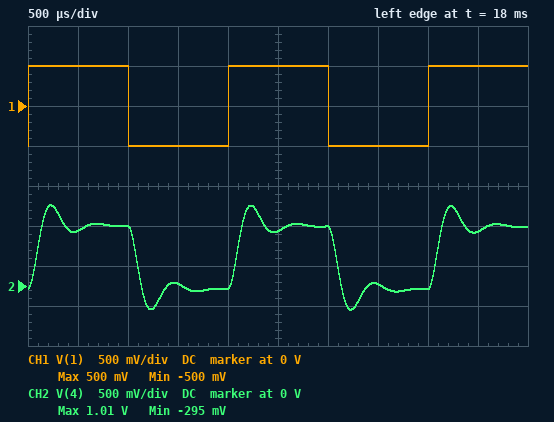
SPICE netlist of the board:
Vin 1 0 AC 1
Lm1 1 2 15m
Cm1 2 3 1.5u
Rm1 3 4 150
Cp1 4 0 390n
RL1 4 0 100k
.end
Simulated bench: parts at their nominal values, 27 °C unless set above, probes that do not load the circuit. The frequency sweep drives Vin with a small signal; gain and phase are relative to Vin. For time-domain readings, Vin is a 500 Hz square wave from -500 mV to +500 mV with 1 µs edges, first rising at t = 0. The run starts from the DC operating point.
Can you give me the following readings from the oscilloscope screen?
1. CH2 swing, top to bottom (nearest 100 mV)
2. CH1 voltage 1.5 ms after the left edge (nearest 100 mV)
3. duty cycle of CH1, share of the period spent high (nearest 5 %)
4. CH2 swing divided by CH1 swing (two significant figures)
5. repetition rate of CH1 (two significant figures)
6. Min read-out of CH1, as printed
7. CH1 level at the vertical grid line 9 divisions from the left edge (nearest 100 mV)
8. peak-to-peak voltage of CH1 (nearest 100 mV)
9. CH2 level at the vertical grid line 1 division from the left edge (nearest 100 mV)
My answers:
1.3 V
-500 mV
50 %
1.3
500 Hz
-500 mV
500 mV
1.0 V
700 mV
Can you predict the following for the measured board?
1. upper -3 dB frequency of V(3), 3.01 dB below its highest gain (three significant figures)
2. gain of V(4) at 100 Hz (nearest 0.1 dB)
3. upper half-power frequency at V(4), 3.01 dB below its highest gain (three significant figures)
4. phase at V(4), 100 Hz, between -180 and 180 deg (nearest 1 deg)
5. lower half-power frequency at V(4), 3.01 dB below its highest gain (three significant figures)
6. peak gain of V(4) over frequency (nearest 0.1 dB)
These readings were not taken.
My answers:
2.97 kHz
-2.0 dB
2.77 kHz
-1 deg
828 Hz
1.8 dB
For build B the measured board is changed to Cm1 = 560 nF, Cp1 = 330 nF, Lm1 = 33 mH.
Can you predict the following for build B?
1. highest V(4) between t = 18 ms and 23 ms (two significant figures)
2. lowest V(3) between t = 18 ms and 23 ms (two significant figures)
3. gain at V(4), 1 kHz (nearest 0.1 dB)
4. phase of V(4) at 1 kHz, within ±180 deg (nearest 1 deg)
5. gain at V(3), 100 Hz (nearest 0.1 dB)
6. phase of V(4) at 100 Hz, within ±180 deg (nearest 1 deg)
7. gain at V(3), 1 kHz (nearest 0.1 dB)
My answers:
890 mV
-450 mV
-1.6 dB
-15 deg
-4.0 dB
0 deg
-1.2 dB
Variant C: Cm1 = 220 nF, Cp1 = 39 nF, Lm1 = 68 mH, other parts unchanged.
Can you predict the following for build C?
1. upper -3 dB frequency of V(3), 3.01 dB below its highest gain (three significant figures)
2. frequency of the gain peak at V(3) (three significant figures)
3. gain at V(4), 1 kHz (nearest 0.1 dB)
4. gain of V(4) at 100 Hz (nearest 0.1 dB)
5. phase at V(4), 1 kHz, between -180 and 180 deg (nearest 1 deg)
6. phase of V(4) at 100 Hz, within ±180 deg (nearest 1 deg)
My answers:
3.53 kHz
3.34 kHz
-0.6 dB
-1.4 dB
-2 deg
3 deg
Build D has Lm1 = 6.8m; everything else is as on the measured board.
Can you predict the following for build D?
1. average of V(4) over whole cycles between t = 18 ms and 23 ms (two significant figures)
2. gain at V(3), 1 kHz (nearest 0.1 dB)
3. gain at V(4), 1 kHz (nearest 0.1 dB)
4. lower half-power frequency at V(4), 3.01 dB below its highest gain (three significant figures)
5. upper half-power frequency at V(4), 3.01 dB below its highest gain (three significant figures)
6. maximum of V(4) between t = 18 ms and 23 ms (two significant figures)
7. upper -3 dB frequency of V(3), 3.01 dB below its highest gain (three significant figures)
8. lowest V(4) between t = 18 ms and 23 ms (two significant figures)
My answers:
360 mV
-1.1 dB
-1.7 dB
1.16 Hz
4.05 kHz
880 mV
4.99 kHz
-170 mV
